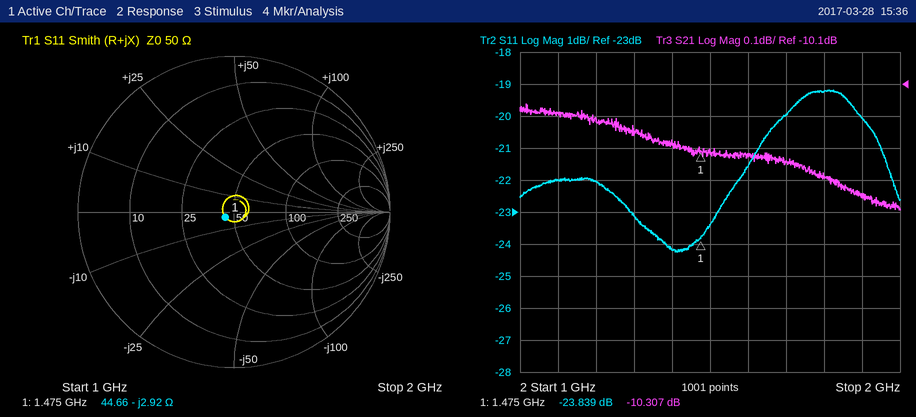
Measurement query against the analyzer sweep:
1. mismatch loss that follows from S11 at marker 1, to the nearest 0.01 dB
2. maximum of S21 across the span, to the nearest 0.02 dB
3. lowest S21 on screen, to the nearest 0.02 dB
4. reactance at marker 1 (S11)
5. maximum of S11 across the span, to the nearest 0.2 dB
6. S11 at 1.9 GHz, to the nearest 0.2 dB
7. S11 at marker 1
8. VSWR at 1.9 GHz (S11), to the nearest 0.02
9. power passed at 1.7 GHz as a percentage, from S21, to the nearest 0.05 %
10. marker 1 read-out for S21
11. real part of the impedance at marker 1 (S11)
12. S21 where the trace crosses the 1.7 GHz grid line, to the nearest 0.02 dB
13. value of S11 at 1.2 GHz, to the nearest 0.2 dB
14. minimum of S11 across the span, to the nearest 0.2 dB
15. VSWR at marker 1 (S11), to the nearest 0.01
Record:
0.02 dB
-10.16 dB
-10.50 dB
-2.92 Ω
-19.2 dB
-20.0 dB
-23.839 dB
1.22
9.25 %
-10.307 dB
44.66 Ω
-10.34 dB
-22.0 dB
-24.2 dB
1.14
